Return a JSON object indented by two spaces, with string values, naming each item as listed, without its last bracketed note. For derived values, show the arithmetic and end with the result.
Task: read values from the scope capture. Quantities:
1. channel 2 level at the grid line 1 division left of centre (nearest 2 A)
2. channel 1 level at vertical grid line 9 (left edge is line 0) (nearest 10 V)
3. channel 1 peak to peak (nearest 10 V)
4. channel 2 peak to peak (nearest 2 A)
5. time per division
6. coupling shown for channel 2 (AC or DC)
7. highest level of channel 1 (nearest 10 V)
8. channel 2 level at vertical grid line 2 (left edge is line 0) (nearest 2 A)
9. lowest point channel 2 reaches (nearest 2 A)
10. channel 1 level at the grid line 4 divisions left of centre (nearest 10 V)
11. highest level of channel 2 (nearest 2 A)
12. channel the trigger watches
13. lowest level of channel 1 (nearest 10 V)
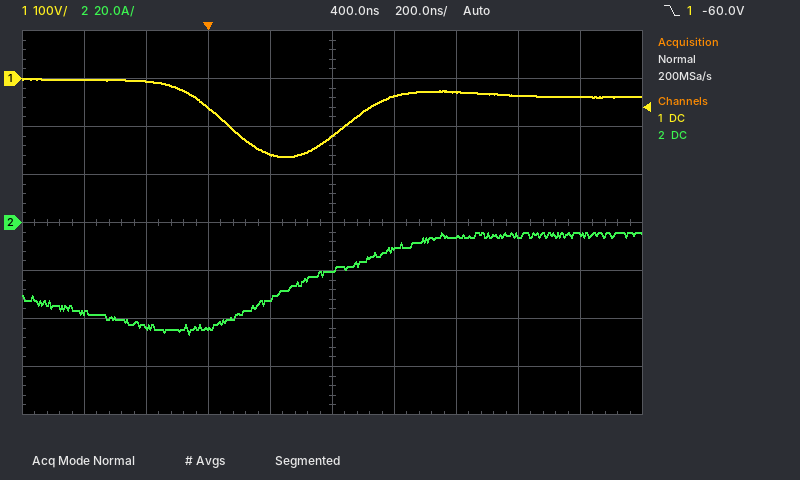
{
  "channel 2 level at the grid line 1 division left of centre": "-32 A",
  "channel 1 level at vertical grid line 9 (left edge is line 0)": "-40 V",
  "channel 1 peak to peak": "0 V − (-160 V) = 160 V",
  "channel 2 peak to peak": "-4 A − (-46 A) = 42 A",
  "time per division": "200 ns",
  "coupling shown for channel 2": "DC",
  "highest level of channel 1": "0 V",
  "channel 2 level at vertical grid line 2 (left edge is line 0)": "-44 A",
  "lowest point channel 2 reaches": "-46 A",
  "channel 1 level at the grid line 4 divisions left of centre": "0 V",
  "highest level of channel 2": "-4 A",
  "channel the trigger watches": "channel 1",
  "lowest level of channel 1": "-160 V"
}
